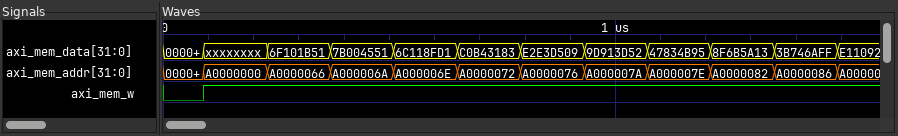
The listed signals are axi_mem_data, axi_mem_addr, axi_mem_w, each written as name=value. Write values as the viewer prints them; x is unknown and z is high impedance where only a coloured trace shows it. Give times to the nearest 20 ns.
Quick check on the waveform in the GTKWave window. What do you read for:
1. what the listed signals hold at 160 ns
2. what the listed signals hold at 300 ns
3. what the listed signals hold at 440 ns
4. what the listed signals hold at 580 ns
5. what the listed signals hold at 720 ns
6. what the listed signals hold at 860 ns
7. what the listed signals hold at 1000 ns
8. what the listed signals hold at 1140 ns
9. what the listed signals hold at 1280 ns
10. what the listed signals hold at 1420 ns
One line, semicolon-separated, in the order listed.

axi_mem_data=xxxxxxxx, axi_mem_addr=A0000000, axi_mem_w=1; axi_mem_data=6F101B51, axi_mem_addr=A0000066, axi_mem_w=1; axi_mem_data=7B004551, axi_mem_addr=A000006A, axi_mem_w=1; axi_mem_data=6C118FD1, axi_mem_addr=A000006E, axi_mem_w=1; axi_mem_data=C0B43183, axi_mem_addr=A0000072, axi_mem_w=1; axi_mem_data=E2E3D509, axi_mem_addr=A0000076, axi_mem_w=1; axi_mem_data=9D913D52, axi_mem_addr=A000007A, axi_mem_w=1; axi_mem_data=47834B95, axi_mem_addr=A000007E, axi_mem_w=1; axi_mem_data=8F6B5A13, axi_mem_addr=A0000082, axi_mem_w=1; axi_mem_data=3B746AFF, axi_mem_addr=A0000086, axi_mem_w=1
